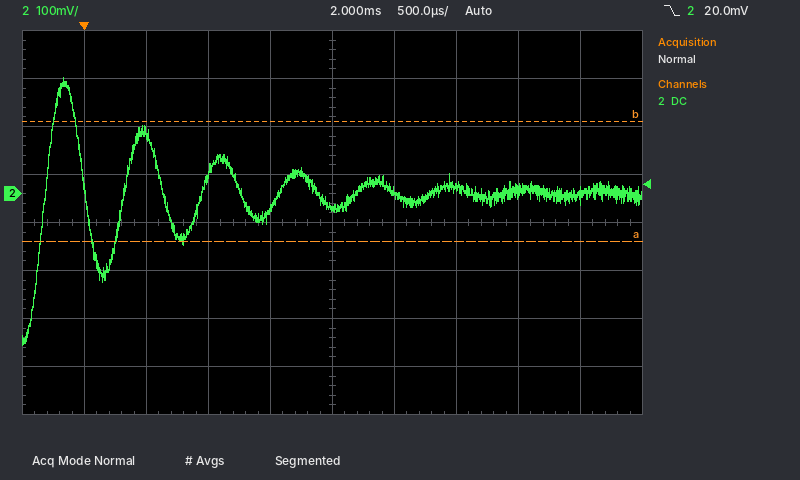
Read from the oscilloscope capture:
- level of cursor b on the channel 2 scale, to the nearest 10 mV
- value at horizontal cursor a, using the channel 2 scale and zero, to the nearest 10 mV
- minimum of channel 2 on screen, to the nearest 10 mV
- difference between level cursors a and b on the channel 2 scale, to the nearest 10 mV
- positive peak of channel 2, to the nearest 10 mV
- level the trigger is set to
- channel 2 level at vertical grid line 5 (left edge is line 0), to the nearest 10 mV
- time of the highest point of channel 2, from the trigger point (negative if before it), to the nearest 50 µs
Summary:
150 mV
-100 mV
-310 mV
250 mV
240 mV
20.0 mV
-30 mV
-150 µs
